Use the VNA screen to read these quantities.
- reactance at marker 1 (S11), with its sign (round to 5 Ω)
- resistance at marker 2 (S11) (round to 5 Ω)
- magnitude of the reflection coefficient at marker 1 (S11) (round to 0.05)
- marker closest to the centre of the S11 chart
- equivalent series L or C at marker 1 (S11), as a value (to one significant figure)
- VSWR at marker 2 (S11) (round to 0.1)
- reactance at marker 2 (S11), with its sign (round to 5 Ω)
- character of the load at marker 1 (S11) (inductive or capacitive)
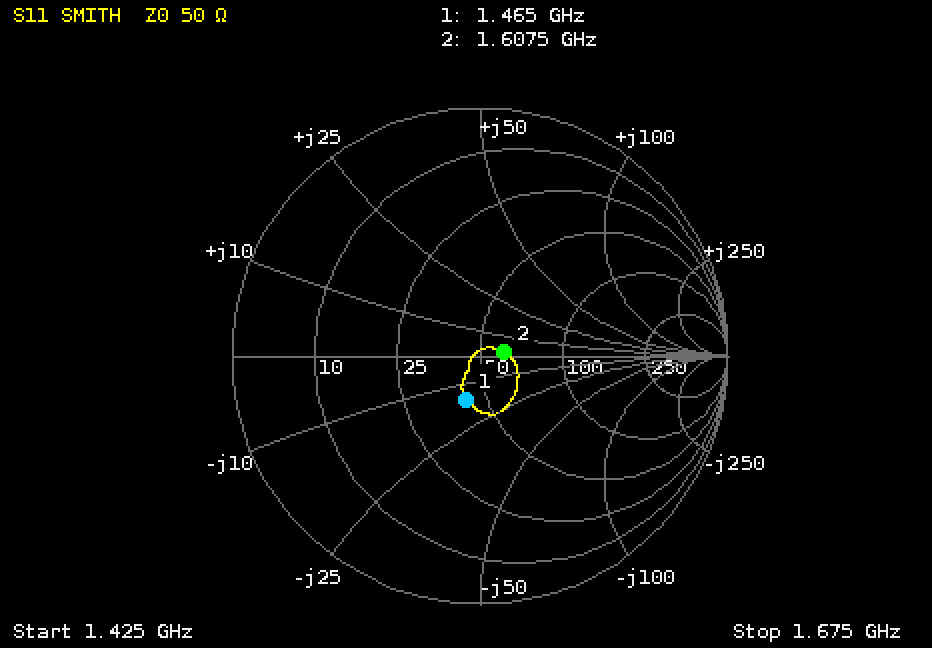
-15 Ω
60 Ω
0.20
marker 2
7 pF
1.2
0 Ω
capacitive
